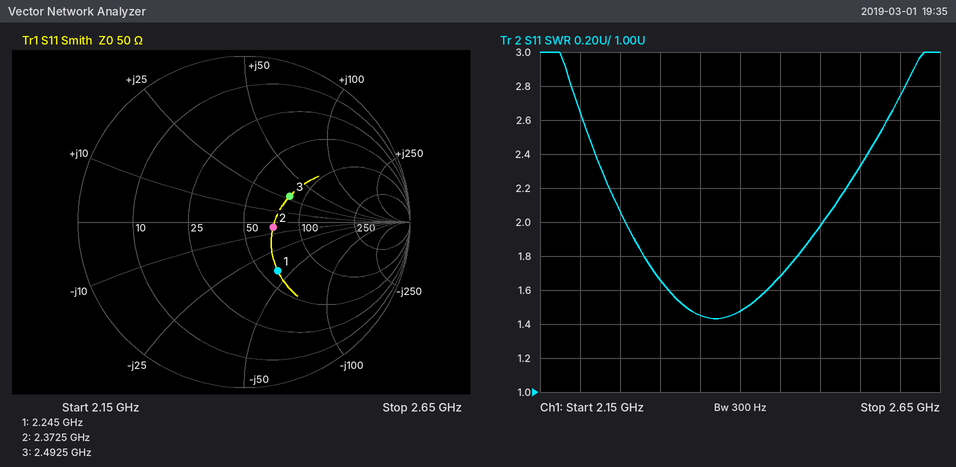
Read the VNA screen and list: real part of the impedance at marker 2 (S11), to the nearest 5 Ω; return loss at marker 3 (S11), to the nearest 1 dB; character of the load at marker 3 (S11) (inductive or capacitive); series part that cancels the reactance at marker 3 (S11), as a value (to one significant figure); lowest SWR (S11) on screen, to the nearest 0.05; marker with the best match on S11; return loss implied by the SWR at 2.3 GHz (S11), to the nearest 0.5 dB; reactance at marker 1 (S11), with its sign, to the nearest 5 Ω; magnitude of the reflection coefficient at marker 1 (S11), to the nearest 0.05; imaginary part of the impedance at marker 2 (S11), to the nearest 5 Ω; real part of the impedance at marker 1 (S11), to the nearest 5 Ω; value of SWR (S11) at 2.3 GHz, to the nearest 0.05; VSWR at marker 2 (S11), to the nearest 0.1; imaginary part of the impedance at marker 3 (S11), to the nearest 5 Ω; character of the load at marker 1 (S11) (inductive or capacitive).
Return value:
70 Ω
10 dB
inductive
2 pF
1.45
marker 2
12.0 dB
-40 Ω
0.35
-5 Ω
60 Ω
1.65
1.4
+30 Ω
capacitive
